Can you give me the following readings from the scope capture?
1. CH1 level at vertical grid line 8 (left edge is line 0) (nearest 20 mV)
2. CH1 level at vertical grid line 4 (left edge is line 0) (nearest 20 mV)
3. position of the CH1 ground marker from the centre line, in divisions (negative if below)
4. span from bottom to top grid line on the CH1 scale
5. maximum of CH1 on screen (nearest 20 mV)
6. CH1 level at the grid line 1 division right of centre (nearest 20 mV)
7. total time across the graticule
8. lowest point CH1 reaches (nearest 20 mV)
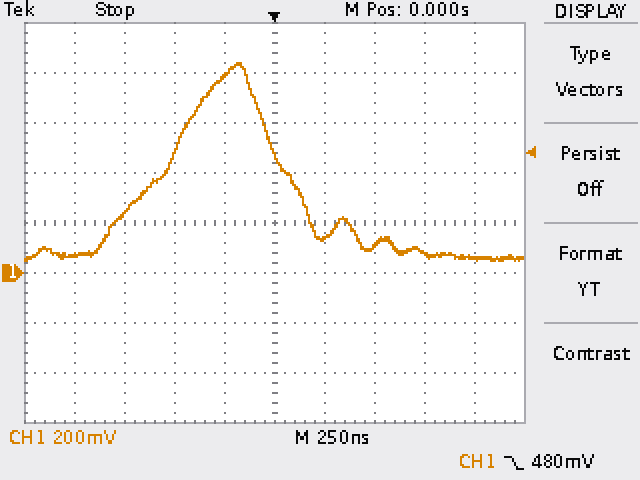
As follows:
80 mV
780 mV
-1.0 div
1.6 V
840 mV
140 mV
2.5 µs
40 mV
